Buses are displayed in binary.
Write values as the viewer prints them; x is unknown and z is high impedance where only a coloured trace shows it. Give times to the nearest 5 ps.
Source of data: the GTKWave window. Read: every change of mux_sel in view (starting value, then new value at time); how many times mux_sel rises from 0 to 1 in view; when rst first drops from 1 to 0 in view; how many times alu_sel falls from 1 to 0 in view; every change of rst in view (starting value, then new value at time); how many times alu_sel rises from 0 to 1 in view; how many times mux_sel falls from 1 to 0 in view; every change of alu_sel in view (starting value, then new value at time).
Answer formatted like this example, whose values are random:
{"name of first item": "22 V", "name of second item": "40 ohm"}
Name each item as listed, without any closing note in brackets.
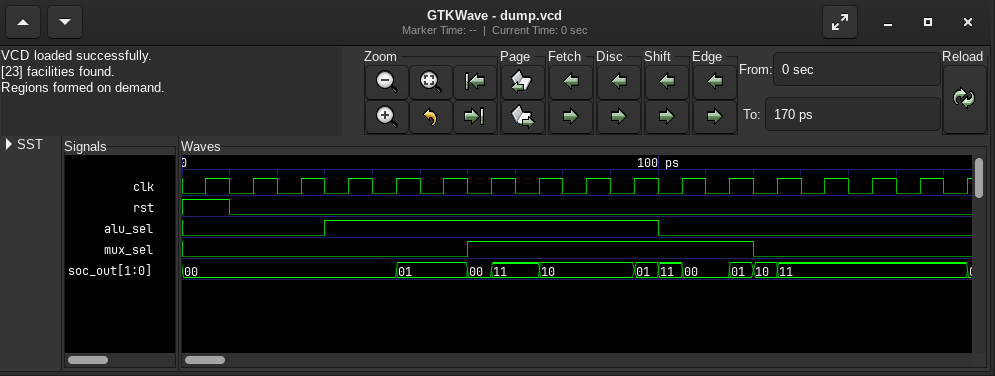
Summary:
{"every change of mux_sel in view": "0, 1 at 60 ps, 0 at 120 ps", "how many times mux_sel rises from 0 to 1 in view": "1", "when rst first drops from 1 to 0 in view": "10 ps", "how many times alu_sel falls from 1 to 0 in view": "1", "every change of rst in view": "1, 0 at 10 ps", "how many times alu_sel rises from 0 to 1 in view": "1", "how many times mux_sel falls from 1 to 0 in view": "1", "every change of alu_sel in view": "0, 1 at 30 ps, 0 at 100 ps"}
